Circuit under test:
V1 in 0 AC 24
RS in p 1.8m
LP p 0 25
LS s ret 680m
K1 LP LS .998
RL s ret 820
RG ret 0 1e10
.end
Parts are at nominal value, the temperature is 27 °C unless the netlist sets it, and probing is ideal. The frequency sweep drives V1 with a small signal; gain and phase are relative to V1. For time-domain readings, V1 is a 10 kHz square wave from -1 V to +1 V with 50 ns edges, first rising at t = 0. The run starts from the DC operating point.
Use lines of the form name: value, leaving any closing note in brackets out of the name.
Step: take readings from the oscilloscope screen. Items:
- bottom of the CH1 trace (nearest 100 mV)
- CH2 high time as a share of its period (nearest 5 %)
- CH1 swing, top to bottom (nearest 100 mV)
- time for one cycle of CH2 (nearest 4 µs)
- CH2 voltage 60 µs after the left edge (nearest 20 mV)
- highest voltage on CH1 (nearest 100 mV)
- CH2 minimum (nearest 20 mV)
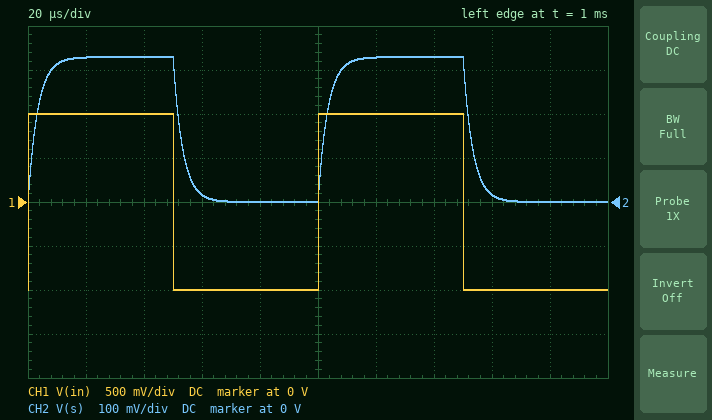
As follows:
bottom of the CH1 trace: -1.0 V
CH2 high time as a share of its period: 50 %
CH1 swing, top to bottom: 2.0 V
time for one cycle of CH2: 100 µs
CH2 voltage 60 µs after the left edge: 20 mV
highest voltage on CH1: 1.0 V
CH2 minimum: 0 V
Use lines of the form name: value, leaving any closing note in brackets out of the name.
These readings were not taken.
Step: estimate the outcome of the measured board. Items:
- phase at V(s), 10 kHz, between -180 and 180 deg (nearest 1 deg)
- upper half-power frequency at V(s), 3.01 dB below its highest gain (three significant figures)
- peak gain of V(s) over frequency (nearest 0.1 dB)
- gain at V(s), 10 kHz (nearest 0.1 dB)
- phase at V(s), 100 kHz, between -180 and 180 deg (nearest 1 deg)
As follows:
phase at V(s), 10 kHz, between -180 and 180 deg: -12 deg
upper half-power frequency at V(s), 3.01 dB below its highest gain: 48.0 kHz
peak gain of V(s) over frequency: -15.7 dB
gain at V(s), 10 kHz: -15.9 dB
phase at V(s), 100 kHz, between -180 and 180 deg: -64 deg
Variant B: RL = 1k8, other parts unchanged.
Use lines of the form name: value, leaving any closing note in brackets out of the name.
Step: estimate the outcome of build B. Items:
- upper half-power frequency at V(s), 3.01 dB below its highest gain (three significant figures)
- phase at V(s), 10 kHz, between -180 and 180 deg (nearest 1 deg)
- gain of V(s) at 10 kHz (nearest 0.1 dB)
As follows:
upper half-power frequency at V(s), 3.01 dB below its highest gain: 105 kHz
phase at V(s), 10 kHz, between -180 and 180 deg: -5 deg
gain of V(s) at 10 kHz: -15.7 dB
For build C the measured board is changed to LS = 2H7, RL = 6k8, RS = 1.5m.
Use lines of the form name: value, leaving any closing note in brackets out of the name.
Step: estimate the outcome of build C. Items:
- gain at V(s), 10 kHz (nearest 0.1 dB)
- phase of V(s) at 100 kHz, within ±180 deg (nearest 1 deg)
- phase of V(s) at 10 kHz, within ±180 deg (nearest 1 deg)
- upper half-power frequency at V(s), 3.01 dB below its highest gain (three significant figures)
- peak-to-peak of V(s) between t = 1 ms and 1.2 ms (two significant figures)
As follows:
gain at V(s), 10 kHz: -9.7 dB
phase of V(s) at 100 kHz, within ±180 deg: -45 deg
phase of V(s) at 10 kHz, within ±180 deg: -6 deg
upper half-power frequency at V(s), 3.01 dB below its highest gain: 100 kHz
peak-to-peak of V(s) between t = 1 ms and 1.2 ms: 660 mV
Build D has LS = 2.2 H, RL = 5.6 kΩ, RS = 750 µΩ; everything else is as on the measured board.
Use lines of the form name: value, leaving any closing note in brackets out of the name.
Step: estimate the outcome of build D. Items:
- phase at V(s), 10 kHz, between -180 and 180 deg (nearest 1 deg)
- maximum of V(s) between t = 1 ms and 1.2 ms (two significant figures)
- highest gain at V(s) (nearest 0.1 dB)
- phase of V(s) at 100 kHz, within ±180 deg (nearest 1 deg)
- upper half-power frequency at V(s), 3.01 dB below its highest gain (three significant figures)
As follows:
phase at V(s), 10 kHz, between -180 and 180 deg: -6 deg
maximum of V(s) between t = 1 ms and 1.2 ms: 590 mV
highest gain at V(s): -10.6 dB
phase of V(s) at 100 kHz, within ±180 deg: -45 deg
upper half-power frequency at V(s), 3.01 dB below its highest gain: 101 kHz
